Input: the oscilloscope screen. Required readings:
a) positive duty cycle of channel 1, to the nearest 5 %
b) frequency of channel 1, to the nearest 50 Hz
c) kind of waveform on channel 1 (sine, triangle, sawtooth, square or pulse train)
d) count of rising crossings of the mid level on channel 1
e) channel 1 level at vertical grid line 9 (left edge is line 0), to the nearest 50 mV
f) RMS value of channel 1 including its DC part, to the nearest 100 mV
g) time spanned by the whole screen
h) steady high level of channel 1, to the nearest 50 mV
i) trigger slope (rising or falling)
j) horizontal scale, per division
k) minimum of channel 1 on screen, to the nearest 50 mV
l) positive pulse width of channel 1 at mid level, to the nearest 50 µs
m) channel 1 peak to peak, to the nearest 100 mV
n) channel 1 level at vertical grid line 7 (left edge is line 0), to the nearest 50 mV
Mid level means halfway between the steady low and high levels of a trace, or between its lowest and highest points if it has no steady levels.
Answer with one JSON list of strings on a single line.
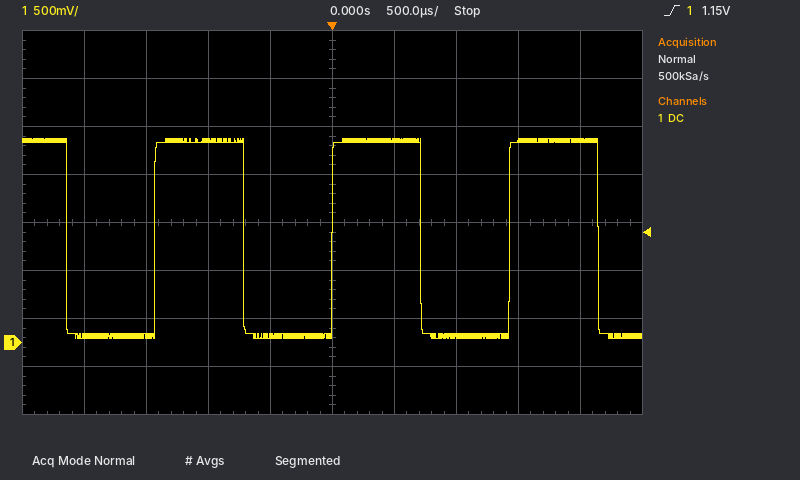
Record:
["50 %", "700 Hz", "square", "3", "2.10 V", "1.5 V", "5 ms", "2.10 V", "rising", "500 µs", "50 mV", "700 µs", "2.10 V", "50 mV"]
